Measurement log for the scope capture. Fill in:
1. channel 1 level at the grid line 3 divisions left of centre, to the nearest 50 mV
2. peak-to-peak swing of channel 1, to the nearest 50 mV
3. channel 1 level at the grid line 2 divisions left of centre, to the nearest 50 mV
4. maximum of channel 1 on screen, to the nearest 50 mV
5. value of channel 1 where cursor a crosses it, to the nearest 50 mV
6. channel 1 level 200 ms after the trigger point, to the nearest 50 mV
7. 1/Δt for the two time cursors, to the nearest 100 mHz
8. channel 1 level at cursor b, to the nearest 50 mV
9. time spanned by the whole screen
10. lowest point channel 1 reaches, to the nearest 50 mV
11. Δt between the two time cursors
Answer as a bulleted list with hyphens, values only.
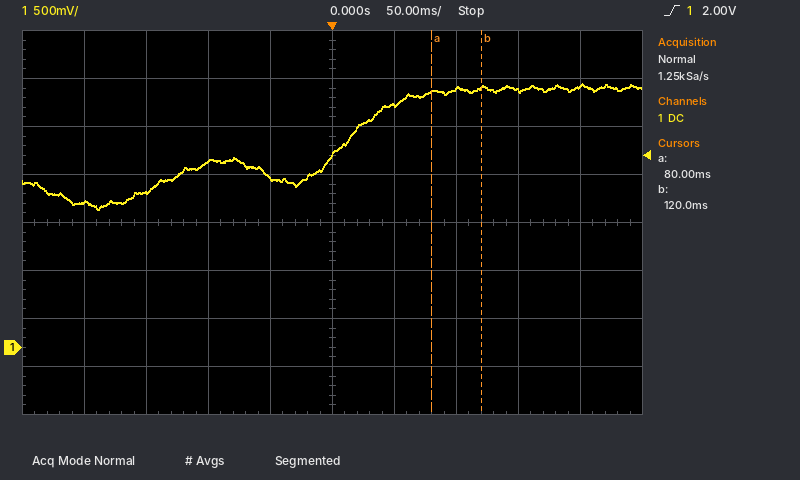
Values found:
- 1.60 V
- 1.30 V
- 1.95 V
- 2.75 V
- 2.65 V
- 2.70 V
- 25.0 Hz
- 2.70 V
- 500 ms
- 1.45 V
- 40 ms
